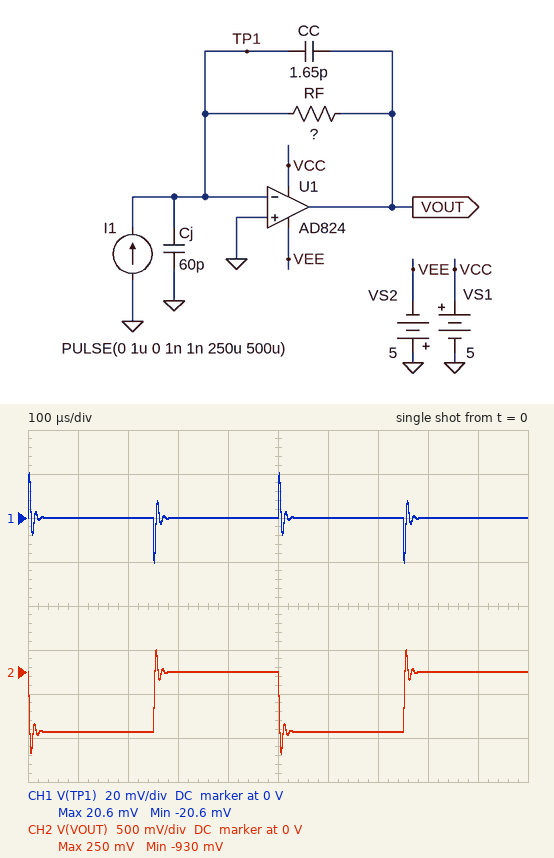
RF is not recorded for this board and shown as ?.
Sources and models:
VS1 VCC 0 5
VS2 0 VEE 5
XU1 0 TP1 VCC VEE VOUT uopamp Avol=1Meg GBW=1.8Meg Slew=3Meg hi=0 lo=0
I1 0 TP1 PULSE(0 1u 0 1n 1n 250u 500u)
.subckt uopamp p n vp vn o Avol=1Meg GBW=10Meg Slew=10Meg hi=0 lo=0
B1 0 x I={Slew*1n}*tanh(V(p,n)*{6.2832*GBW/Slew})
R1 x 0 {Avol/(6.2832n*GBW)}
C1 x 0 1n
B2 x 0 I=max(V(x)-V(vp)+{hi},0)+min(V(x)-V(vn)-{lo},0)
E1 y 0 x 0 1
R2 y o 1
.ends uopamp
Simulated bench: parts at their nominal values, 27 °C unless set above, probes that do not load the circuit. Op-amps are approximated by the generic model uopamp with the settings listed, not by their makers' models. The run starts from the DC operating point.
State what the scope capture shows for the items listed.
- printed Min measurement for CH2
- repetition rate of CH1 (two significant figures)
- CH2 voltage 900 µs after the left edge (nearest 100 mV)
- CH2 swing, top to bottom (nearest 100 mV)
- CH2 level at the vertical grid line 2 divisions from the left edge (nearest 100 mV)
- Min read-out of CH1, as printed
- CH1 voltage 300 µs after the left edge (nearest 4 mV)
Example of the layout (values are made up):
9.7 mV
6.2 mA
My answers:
-930 mV
2.0 kHz
0 V
1.2 V
-700 mV
-20.6 mV
0 V
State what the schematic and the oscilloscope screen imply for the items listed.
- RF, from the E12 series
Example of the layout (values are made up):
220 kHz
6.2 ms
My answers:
680 kΩ
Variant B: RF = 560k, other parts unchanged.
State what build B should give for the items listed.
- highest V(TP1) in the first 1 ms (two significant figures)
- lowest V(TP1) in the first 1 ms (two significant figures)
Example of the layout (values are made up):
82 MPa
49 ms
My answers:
19 mV
-19 mV
